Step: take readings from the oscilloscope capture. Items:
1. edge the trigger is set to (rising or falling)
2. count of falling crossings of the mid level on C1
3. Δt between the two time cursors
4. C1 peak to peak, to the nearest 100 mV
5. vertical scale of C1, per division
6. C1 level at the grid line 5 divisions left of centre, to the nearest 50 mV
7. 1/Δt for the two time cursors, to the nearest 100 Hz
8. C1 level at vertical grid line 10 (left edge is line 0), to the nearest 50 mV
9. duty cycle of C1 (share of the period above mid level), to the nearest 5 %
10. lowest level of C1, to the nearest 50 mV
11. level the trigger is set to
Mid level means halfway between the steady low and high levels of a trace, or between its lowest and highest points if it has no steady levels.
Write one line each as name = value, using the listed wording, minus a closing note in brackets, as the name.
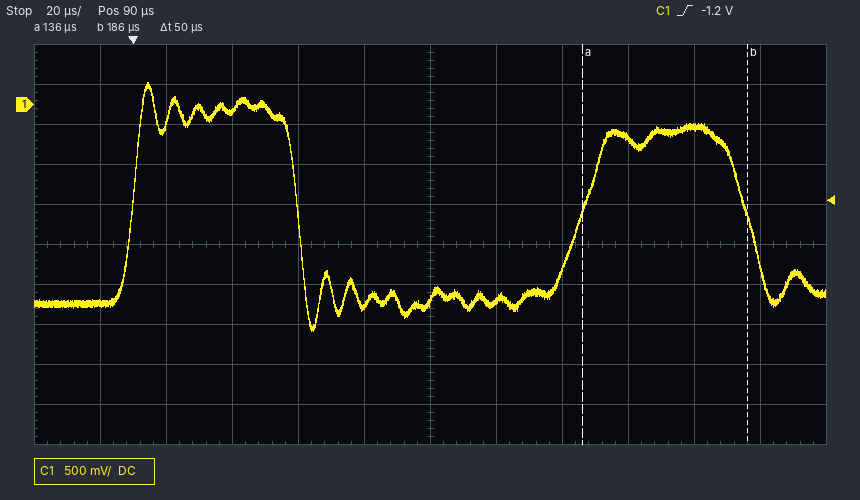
edge the trigger is set to = rising
count of falling crossings of the mid level on C1 = 2
Δt between the two time cursors = 50 µs
C1 peak to peak, to the nearest 100 mV = 3.10 V
vertical scale of C1, per division = 500 mV
C1 level at the grid line 5 divisions left of centre, to the nearest 50 mV = -2.50 V
1/Δt for the two time cursors, to the nearest 100 Hz = 20.0 kHz
C1 level at vertical grid line 10 (left edge is line 0), to the nearest 50 mV = -300 mV
duty cycle of C1 (share of the period above mid level), to the nearest 5 % = 35 %
lowest level of C1, to the nearest 50 mV = -2.85 V
level the trigger is set to = -1.2 V
